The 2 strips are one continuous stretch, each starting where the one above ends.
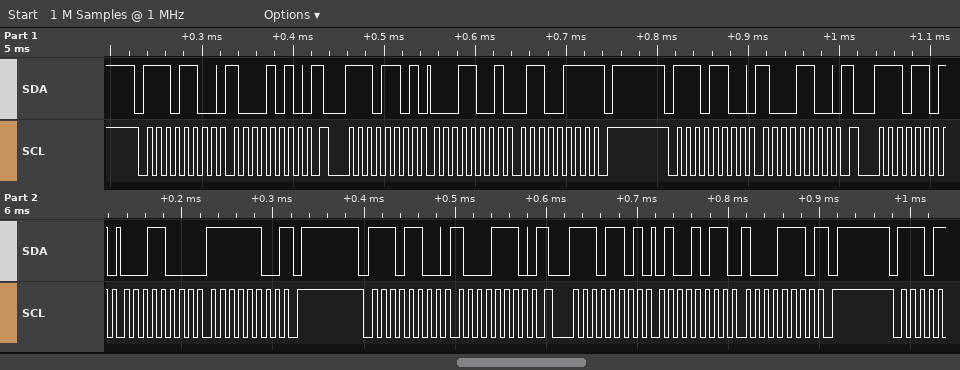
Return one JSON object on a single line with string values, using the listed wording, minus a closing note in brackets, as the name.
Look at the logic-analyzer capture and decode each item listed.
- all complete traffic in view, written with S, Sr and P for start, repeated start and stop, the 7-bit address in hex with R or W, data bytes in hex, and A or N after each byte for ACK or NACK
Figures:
{"all complete traffic in view, written with S, Sr and P for start, repeated start and stop, the 7-bit address in hex with R or W, data bytes in hex, and A or N after each byte for ACK or NACK": "S 76W A 8A A Sr 76R A 19 A 67 N P S 76W A 8C A Sr 76R A 18 A FC N P S 76W A 8E A Sr 76R A 4B A 8E N P"}
